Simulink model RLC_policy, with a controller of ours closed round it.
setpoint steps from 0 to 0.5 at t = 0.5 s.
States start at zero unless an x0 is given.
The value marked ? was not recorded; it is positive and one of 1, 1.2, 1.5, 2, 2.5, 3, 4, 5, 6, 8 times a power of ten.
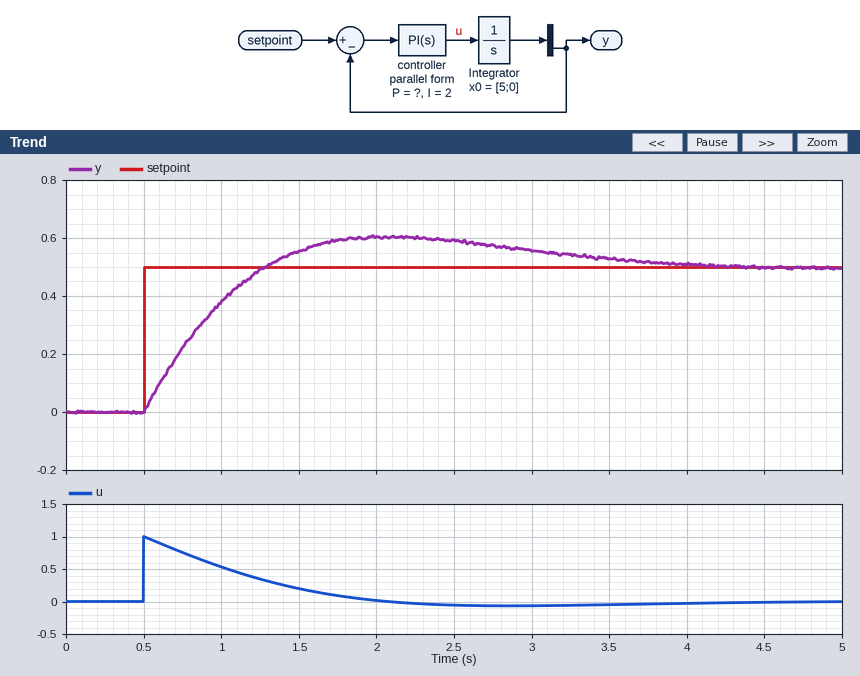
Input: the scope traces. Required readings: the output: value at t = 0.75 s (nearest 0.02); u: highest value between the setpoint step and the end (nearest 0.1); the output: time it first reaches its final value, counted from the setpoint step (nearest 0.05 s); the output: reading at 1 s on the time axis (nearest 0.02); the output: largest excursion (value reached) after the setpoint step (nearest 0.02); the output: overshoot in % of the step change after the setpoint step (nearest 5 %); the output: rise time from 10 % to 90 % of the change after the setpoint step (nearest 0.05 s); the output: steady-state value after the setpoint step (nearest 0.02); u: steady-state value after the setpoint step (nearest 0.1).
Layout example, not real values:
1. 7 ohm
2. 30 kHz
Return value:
1. 0.22
2. 1.0
3. 0.80 s
4. 0.38
5. 0.60
6. 20 %
7. 0.60 s
8. 0.50
9. 0.0
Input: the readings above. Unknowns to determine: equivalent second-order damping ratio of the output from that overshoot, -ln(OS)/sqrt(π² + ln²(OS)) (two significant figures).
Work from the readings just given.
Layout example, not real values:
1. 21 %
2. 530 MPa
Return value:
1. 0.46
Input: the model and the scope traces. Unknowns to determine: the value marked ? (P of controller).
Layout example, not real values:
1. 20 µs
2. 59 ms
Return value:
1. 2
